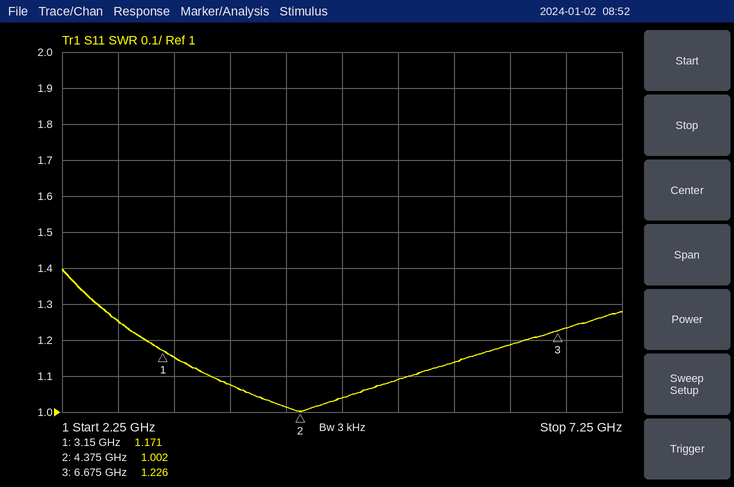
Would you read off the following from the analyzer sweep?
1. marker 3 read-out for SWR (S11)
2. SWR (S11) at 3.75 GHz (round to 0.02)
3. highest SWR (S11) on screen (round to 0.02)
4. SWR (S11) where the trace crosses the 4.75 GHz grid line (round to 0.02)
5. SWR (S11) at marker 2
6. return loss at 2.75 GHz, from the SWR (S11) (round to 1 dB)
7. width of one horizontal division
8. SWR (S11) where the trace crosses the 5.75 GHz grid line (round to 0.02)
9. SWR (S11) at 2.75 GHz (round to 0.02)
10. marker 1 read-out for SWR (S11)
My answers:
1.226
1.08
1.40
1.04
1.002
19 dB
500 MHz
1.14
1.26
1.171
